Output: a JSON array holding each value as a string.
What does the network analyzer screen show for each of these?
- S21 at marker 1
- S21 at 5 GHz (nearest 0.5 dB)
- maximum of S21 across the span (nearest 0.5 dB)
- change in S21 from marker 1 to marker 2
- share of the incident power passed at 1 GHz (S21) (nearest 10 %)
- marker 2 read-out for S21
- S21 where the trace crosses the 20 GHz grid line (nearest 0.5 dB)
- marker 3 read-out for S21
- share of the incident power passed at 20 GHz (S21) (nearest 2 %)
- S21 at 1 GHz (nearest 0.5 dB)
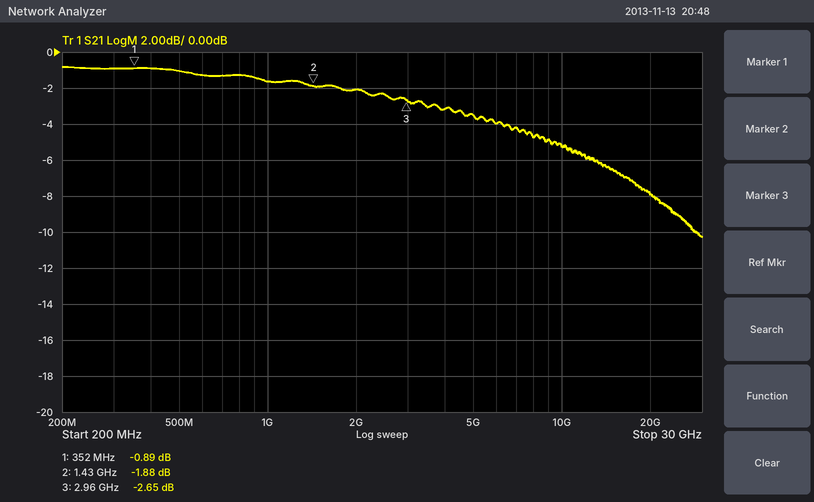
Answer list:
["-0.89 dB", "-3.5 dB", "-1.0 dB", "-0.99 dB", "70 %", "-1.88 dB", "-8.0 dB", "-2.65 dB", "16 %", "-1.5 dB"]
